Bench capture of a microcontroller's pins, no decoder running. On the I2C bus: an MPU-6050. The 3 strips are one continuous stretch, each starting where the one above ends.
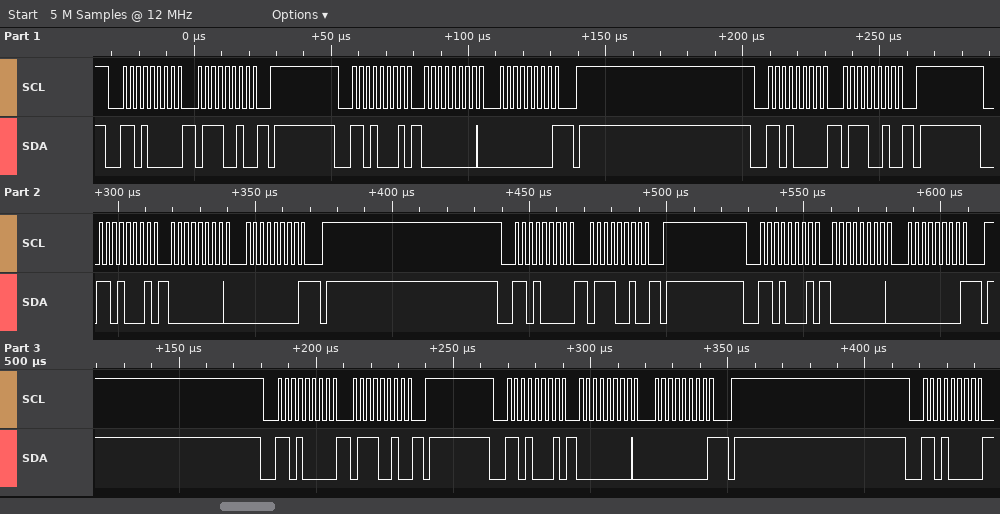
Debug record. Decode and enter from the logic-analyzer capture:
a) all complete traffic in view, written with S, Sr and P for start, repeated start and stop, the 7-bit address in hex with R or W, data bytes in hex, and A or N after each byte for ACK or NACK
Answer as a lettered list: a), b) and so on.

a) S 68W A 72 A P S 68R A 00 A 00 N P S 68W A 72 A P S 68R A 00 A 00 N P S 68W A 72 A P S 68R A 00 A 00 N P S 68W A 72 A P S 68R A 00 A 00 N P S 68W A
